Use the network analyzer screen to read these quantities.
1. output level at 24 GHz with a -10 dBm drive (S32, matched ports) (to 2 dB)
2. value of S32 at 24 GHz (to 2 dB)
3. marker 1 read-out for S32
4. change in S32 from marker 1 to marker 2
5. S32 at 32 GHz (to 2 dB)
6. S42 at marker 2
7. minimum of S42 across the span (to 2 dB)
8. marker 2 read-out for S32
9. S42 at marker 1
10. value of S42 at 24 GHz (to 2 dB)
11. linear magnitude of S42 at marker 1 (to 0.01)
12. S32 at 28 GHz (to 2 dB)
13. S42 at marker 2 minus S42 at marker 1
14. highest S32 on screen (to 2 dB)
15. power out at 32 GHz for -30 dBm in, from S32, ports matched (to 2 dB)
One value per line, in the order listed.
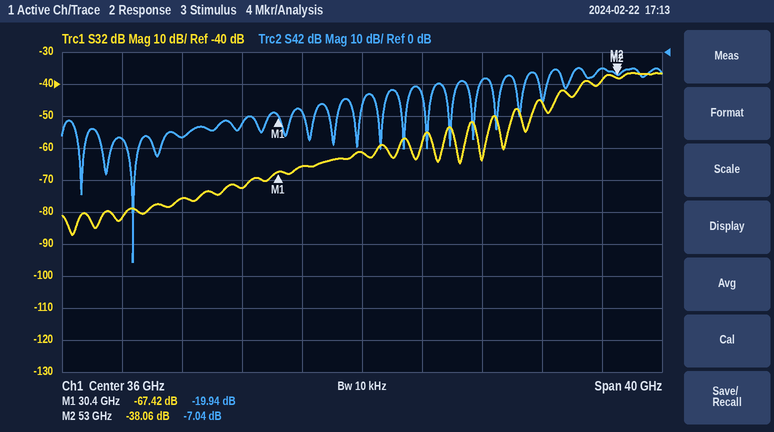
-86 dBm
-76 dB
-67.42 dB
29.36 dB
-66 dB
-7.04 dB
-66 dB
-38.06 dB
-19.94 dB
-26 dB
0.10
-72 dB
12.90 dB
-36 dB
-96 dBm
